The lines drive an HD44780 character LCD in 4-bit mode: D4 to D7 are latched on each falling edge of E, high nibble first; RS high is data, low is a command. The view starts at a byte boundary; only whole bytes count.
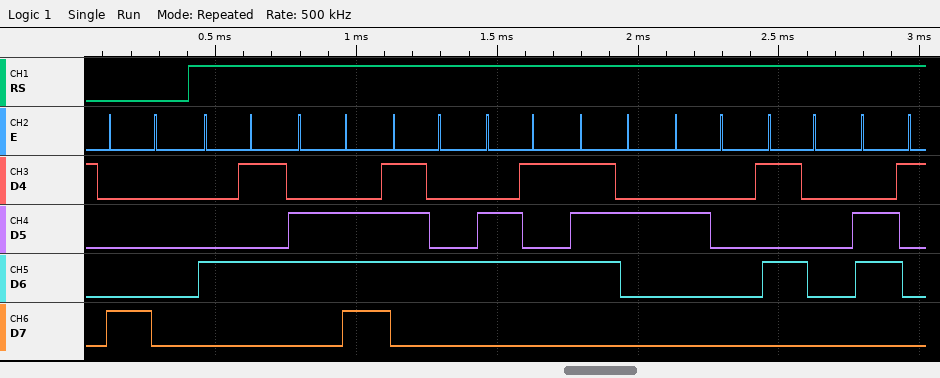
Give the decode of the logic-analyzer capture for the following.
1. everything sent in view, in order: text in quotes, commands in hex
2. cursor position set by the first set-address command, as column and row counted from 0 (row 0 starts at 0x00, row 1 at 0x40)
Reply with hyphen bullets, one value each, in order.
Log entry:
- 0x80 "Enter Pa"
- column 0, row 0
